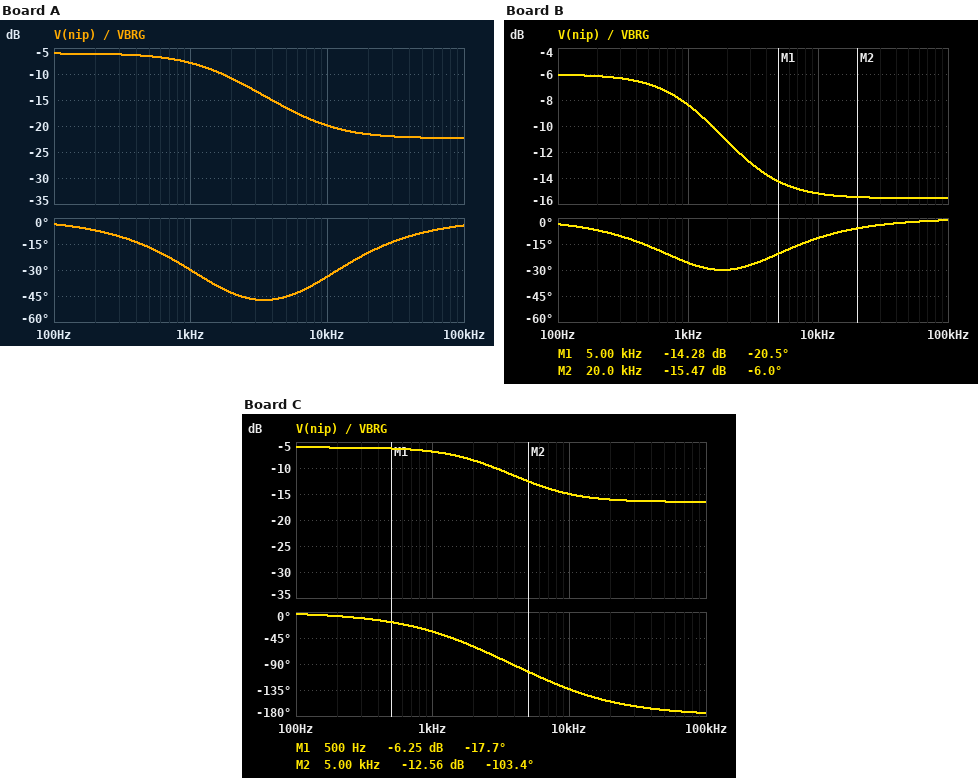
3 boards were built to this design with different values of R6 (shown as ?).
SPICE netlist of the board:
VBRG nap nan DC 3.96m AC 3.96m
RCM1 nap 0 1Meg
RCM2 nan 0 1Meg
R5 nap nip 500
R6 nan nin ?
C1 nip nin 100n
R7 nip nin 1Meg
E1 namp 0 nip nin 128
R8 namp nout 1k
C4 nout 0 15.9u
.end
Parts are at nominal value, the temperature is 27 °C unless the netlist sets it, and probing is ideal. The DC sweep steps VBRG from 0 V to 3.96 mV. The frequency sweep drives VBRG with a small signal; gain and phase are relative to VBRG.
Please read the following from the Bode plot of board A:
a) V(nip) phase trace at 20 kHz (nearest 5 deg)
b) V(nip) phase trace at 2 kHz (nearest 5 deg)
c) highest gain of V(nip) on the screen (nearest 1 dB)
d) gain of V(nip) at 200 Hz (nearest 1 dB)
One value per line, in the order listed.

-20 deg
-45 deg
-6 dB
-6 dB
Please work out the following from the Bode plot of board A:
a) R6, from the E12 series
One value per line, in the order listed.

680 Ω
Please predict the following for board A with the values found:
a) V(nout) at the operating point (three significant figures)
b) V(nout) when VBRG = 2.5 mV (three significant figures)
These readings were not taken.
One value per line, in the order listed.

506 mV
320 mV
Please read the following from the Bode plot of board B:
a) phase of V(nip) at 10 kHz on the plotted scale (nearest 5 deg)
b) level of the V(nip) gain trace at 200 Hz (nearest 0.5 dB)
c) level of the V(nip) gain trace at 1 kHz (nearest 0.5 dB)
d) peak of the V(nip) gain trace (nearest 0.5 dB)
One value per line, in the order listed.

-10 deg
-6.0 dB
-8.5 dB
-6.0 dB
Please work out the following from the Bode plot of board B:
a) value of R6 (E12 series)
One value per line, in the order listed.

1 kΩ
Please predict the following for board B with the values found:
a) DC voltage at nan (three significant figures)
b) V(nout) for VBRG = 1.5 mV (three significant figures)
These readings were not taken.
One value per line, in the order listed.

-1.98 mV
192 mV
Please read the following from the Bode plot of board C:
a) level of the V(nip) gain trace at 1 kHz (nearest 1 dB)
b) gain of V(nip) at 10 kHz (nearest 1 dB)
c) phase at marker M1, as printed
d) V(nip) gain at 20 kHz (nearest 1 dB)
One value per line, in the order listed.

-7 dB
-15 dB
-17.7 deg
-16 dB
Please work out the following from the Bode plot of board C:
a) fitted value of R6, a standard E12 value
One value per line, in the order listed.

270 Ω
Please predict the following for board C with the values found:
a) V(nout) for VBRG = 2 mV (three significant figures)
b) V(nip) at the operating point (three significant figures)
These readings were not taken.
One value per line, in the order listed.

256 mV
1.98 mV
